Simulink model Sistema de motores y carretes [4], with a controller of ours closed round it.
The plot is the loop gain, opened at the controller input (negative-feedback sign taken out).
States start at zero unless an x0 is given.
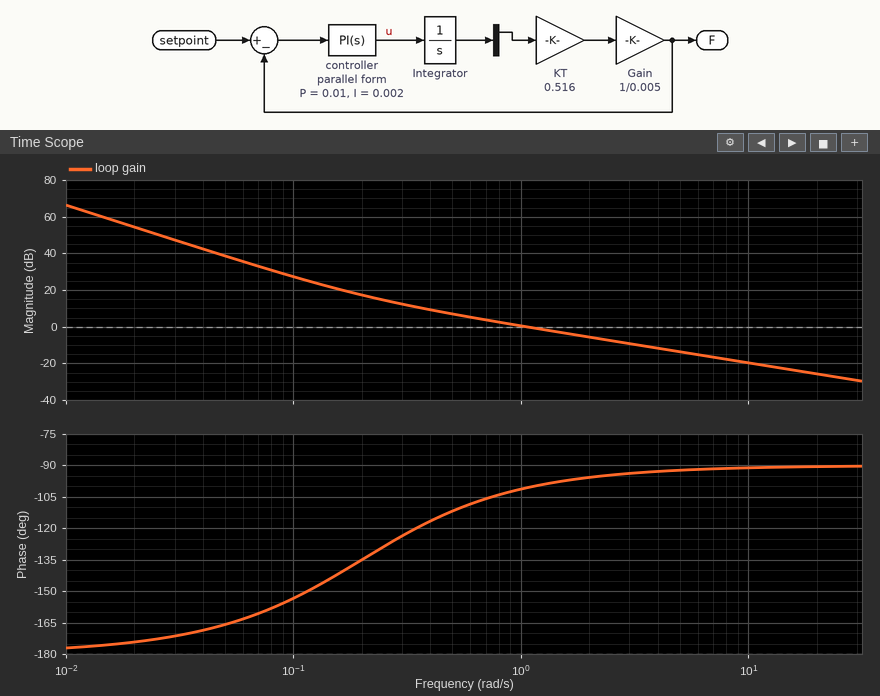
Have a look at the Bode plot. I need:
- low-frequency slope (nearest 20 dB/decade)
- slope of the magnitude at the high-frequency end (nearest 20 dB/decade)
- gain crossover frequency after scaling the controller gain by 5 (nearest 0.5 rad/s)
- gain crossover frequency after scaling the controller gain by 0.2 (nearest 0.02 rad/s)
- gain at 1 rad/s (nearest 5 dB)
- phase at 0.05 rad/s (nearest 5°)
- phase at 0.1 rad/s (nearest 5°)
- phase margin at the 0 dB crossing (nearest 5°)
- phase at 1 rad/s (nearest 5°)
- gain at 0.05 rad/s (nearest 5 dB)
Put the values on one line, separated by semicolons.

-40 dB/decade; -20 dB/decade; 5.0 rad/s; 0.26 rad/s; 0 dB; -165°; -155°; 80°; -100°; 40 dB
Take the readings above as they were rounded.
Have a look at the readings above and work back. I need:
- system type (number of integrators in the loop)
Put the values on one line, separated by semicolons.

2
